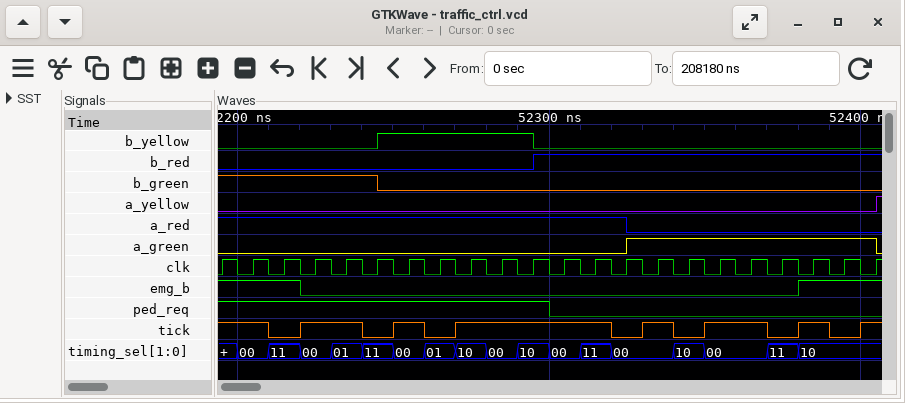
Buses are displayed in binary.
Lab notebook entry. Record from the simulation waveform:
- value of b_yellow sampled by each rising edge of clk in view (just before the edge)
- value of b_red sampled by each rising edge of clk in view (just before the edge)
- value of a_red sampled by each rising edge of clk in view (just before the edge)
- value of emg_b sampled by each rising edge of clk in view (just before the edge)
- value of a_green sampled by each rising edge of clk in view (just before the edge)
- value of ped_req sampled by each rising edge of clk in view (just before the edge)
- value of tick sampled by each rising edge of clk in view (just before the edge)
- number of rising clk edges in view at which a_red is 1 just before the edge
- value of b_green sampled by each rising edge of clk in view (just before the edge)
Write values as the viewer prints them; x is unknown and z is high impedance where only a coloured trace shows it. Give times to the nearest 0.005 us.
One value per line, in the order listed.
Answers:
0 0 0 0 0 0 1 1 1 1 1 0 0 0 0 0 0 0 0 0 0 0
0 0 0 0 0 0 0 0 0 0 0 1 1 1 1 1 1 1 1 1 1 1
1 1 1 1 1 1 1 1 1 1 1 1 1 1 0 0 0 0 0 0 0 0
1 1 1 0 0 0 0 0 0 0 0 0 0 0 0 0 0 0 0 1 1 1
0 0 0 0 0 0 0 0 0 0 0 0 0 0 1 1 1 1 1 1 1 1
1 1 1 1 1 1 1 1 1 1 1 0 0 0 0 0 0 0 0 0 0 0
1 1 0 1 1 0 1 0 1 1 1 1 1 0 1 0 1 1 0 1 0 1
14
1 1 1 1 1 1 0 0 0 0 0 0 0 0 0 0 0 0 0 0 0 0
